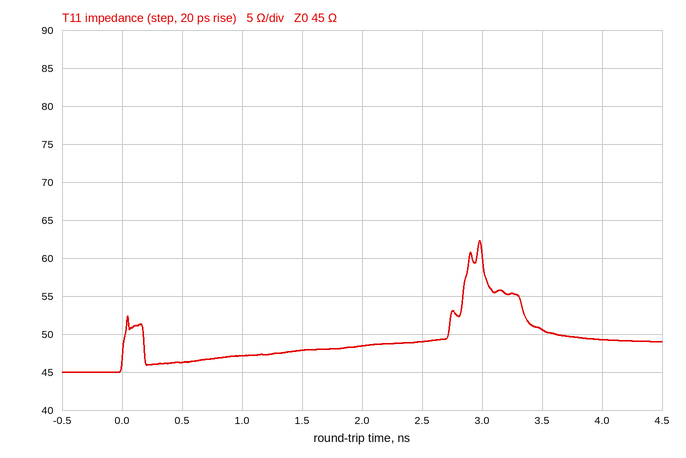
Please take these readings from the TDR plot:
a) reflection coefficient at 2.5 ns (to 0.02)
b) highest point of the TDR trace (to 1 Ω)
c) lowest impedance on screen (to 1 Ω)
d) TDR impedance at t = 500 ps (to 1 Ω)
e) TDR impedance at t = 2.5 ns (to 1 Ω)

+0.04
62 Ω
45 Ω
46 Ω
49 Ω
